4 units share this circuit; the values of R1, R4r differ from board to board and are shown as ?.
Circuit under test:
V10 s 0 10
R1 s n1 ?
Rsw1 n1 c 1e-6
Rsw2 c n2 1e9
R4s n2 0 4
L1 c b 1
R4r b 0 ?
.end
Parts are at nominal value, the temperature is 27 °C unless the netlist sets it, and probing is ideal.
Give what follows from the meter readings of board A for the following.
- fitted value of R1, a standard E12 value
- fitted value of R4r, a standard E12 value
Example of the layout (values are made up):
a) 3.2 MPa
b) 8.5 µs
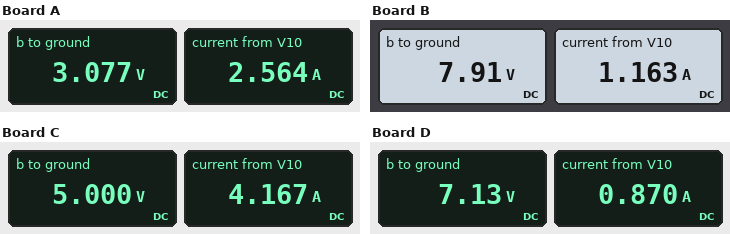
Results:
a) 2.7 Ω
b) 1.2 Ω
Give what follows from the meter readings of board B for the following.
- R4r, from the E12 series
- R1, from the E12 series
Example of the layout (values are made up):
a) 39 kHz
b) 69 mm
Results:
a) 6.8 Ω
b) 1.8 Ω
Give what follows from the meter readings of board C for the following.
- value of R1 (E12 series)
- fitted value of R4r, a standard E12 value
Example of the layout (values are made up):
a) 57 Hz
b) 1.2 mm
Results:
a) 1.2 Ω
b) 1.2 Ω
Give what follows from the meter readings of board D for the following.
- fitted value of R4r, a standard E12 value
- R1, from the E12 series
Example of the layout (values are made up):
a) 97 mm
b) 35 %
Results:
a) 8.2 Ω
b) 3.3 Ω
